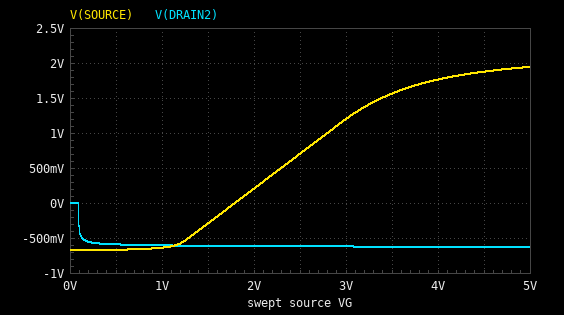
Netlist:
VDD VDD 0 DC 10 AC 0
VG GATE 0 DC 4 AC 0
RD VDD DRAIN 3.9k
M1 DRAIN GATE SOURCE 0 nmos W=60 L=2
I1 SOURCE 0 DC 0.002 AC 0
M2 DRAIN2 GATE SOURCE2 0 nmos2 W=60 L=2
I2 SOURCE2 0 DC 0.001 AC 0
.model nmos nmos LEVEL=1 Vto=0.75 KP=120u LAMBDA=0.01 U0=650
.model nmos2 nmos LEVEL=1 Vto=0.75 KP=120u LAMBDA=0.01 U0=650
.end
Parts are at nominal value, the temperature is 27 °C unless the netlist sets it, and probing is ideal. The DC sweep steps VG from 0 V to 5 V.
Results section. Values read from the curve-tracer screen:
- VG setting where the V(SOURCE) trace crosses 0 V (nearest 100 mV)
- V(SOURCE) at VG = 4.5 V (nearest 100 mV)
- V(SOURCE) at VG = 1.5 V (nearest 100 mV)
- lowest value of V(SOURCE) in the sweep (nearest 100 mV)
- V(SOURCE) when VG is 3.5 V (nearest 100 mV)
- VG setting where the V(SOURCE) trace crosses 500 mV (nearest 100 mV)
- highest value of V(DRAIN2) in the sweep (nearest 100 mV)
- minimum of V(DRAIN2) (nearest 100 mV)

1.8 V
1.9 V
-300 mV
-700 mV
1.6 V
2.3 V
0 V
-600 mV
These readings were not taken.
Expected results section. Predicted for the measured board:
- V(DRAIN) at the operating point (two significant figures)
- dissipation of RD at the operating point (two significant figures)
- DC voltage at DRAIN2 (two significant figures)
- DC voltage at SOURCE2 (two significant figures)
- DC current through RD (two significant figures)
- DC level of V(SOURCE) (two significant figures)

2.2 V
16 mW
-620 mV
-650 mV
2.0 mA
1.8 V
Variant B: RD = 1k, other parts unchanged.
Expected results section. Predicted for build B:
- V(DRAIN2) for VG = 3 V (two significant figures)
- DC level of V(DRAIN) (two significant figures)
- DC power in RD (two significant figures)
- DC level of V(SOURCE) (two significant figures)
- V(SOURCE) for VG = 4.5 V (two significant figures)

-620 mV
8.0 V
4.0 mW
2.2 V
2.7 V
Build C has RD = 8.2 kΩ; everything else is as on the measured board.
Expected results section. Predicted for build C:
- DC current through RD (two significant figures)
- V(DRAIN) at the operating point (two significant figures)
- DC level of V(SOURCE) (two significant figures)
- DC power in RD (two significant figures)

1.3 mA
-550 mV
-650 mV
14 mW
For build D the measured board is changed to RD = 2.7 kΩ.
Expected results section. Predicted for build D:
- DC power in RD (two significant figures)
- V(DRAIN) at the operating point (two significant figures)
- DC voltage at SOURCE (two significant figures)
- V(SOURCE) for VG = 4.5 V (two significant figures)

11 mW
4.6 V
2.2 V
2.7 V
